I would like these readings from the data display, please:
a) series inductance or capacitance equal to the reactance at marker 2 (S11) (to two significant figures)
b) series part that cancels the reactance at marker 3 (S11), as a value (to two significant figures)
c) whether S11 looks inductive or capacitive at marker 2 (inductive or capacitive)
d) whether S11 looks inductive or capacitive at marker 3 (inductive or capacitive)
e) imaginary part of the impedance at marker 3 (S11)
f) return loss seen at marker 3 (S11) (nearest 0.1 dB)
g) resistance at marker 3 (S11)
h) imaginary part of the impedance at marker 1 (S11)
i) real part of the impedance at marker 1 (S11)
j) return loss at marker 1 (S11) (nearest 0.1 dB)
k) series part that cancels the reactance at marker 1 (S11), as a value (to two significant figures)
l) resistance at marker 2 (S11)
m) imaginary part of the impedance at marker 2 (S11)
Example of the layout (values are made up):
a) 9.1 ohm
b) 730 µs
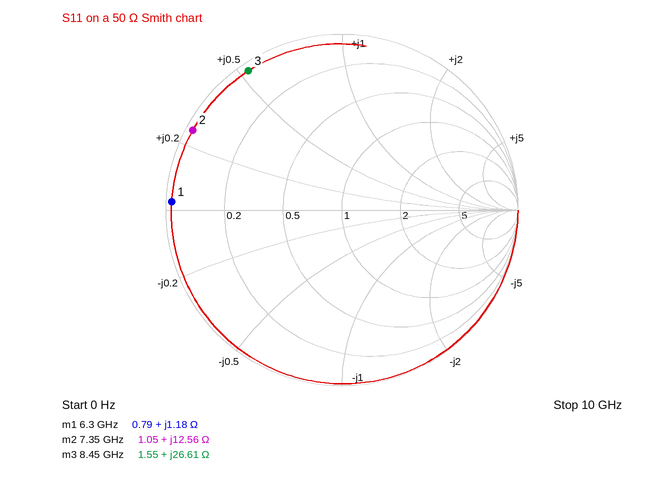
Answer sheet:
a) 270 pH
b) 710 fF
c) inductive
d) inductive
e) +26.61 Ω
f) 0.4 dB
g) 1.55 Ω
h) +1.18 Ω
i) 0.79 Ω
j) 0.3 dB
k) 21 pF
l) 1.05 Ω
m) +12.56 Ω
